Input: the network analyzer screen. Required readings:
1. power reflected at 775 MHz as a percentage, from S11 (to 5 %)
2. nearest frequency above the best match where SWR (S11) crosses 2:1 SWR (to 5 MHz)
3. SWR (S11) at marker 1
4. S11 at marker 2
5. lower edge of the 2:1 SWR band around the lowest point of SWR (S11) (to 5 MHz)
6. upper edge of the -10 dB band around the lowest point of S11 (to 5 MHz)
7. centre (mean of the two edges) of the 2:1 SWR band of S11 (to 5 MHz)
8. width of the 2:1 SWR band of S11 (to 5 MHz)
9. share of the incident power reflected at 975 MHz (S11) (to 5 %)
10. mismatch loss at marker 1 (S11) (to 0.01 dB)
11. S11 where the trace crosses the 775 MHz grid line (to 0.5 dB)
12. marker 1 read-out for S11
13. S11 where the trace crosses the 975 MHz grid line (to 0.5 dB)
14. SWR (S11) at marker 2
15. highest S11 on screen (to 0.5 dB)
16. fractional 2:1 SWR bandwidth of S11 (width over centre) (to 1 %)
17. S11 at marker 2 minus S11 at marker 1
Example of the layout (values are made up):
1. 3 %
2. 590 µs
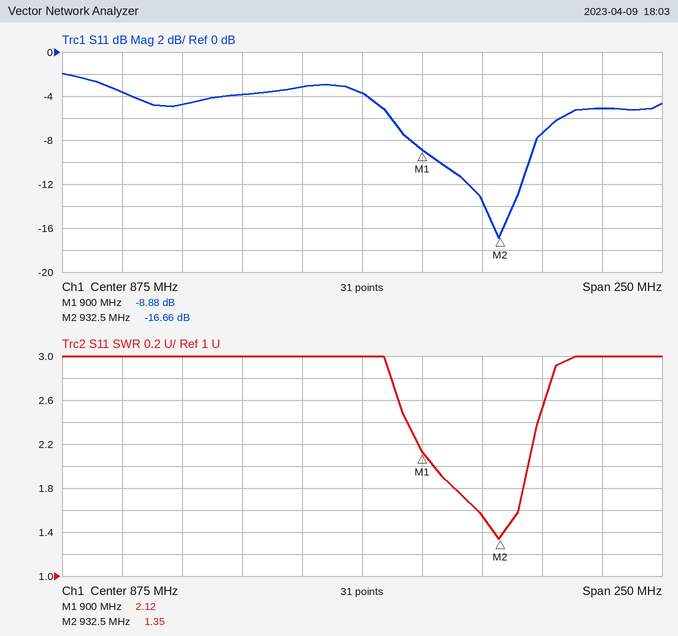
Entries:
1. 45 %
2. 945 MHz
3. 2.12
4. -16.66 dB
5. 905 MHz
6. 945 MHz
7. 925 MHz
8. 40 MHz
9. 30 %
10. 0.60 dB
11. -3.5 dB
12. -8.88 dB
13. -5.0 dB
14. 1.35
15. -2.0 dB
16. 4 %
17. -7.78 dB
